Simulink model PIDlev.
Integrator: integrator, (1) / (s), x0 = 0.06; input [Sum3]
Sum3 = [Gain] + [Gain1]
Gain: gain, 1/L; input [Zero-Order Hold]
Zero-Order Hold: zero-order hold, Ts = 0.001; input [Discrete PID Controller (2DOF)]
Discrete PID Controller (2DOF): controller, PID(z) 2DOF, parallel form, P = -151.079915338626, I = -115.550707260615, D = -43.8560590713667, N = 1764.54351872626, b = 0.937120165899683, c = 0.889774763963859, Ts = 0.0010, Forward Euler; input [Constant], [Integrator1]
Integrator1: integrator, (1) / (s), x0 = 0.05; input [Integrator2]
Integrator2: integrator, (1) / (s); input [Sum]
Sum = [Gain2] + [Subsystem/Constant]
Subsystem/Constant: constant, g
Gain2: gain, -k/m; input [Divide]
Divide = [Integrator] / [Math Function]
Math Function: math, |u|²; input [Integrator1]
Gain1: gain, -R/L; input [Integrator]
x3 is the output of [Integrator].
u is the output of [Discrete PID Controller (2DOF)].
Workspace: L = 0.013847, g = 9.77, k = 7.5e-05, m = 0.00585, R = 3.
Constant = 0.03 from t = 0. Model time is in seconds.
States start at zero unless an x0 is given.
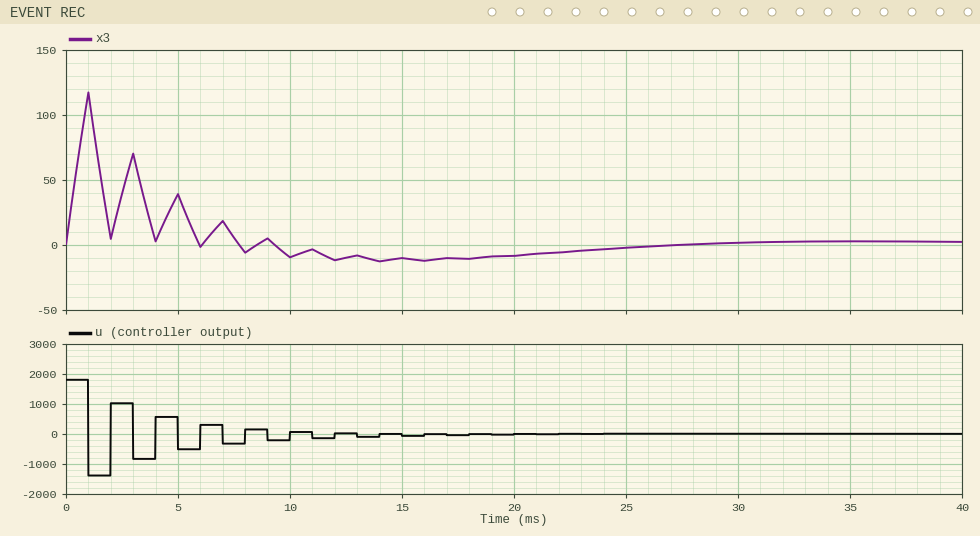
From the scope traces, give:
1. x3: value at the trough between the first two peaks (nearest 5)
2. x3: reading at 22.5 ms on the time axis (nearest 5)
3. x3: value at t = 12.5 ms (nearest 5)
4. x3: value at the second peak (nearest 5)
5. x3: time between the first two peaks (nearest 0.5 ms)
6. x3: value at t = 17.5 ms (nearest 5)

5
-5
-10
70
2.0 ms
-10
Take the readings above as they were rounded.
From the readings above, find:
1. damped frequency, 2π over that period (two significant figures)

3.1 rad/ms
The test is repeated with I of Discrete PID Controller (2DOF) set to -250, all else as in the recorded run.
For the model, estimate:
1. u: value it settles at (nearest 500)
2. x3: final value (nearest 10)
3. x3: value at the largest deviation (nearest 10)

0
0
120
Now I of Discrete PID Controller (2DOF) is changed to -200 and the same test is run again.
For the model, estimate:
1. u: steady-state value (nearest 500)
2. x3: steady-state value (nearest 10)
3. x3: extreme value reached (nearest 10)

0
0
120
